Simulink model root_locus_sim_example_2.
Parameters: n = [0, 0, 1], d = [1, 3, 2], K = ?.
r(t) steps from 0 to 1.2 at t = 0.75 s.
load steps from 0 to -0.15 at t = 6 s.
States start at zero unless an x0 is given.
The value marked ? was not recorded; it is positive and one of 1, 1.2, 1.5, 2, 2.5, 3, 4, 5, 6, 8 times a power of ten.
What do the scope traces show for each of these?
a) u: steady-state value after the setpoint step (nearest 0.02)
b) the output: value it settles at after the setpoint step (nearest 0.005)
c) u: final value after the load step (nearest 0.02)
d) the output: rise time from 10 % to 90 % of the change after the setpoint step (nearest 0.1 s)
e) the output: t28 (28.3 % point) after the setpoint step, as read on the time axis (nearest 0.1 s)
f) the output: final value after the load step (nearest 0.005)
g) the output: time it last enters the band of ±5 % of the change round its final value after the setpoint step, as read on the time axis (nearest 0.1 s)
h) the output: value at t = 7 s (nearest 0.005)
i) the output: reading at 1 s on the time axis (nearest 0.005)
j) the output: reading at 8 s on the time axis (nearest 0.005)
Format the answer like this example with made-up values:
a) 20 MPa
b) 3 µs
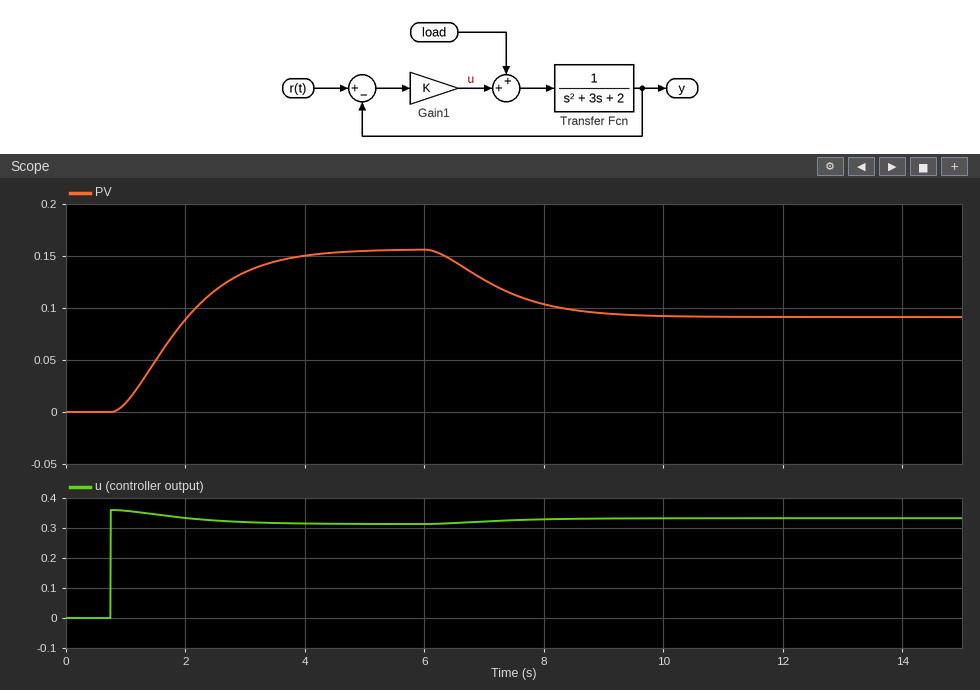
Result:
a) 0.32
b) 0.155
c) 0.34
d) 2.2 s
e) 1.4 s
f) 0.090
g) 3.8 s
h) 0.125
i) 0.010
j) 0.105
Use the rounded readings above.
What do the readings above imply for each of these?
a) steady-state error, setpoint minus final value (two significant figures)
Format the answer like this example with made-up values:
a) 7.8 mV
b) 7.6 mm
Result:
a) 1.0
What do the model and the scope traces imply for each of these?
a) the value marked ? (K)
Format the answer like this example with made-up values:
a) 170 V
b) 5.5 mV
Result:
a) 0.3
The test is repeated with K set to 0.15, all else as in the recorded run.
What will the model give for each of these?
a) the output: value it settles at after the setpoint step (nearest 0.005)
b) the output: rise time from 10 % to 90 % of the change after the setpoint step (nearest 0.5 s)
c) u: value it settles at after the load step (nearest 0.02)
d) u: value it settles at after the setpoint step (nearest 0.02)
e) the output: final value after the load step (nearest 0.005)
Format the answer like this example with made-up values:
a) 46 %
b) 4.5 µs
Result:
a) 0.085
b) 2.5 s
c) 0.18
d) 0.16
e) 0.015
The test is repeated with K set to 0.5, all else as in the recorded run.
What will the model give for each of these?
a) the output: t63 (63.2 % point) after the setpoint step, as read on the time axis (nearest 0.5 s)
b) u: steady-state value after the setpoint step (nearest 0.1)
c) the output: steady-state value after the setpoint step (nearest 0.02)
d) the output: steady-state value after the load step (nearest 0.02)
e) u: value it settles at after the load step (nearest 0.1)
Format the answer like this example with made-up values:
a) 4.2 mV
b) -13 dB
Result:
a) 2.0 s
b) 0.5
c) 0.24
d) 0.18
e) 0.5
